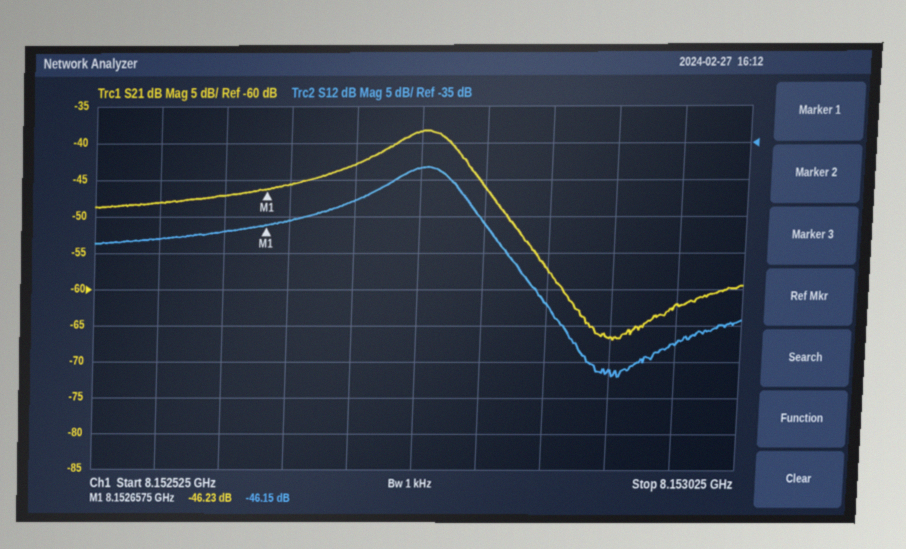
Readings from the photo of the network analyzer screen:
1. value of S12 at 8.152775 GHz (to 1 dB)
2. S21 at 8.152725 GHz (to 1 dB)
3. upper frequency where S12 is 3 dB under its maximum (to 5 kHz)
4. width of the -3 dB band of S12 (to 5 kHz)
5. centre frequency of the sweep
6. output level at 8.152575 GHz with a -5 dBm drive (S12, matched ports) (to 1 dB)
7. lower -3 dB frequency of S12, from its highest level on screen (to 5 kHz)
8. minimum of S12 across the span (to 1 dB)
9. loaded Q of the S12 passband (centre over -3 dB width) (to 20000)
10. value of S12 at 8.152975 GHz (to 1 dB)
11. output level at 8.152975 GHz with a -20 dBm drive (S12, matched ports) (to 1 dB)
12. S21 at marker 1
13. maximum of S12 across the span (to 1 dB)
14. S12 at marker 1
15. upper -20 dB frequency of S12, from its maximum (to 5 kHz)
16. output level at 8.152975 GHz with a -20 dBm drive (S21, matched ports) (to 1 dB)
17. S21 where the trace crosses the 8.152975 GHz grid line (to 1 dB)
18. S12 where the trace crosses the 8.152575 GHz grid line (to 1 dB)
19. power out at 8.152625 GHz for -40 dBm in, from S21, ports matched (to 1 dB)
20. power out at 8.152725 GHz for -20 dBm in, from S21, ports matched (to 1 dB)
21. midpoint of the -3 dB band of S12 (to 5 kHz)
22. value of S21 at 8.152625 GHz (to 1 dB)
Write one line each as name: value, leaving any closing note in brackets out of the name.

value of S12 at 8.152775 GHz: -38 dB
S21 at 8.152725 GHz: -43 dB
upper frequency where S12 is 3 dB under its maximum: 8.152805 GHz
width of the -3 dB band of S12: 60 kHz
centre frequency of the sweep: 8.152775 GHz
output level at 8.152575 GHz with a -5 dBm drive (S12, matched ports): -53 dBm
lower -3 dB frequency of S12, from its highest level on screen: 8.152745 GHz
minimum of S12 across the span: -67 dB
loaded Q of the S12 passband (centre over -3 dB width): 140000
value of S12 at 8.152975 GHz: -63 dB
output level at 8.152975 GHz with a -20 dBm drive (S12, matched ports): -83 dBm
S21 at marker 1: -46.23 dB
maximum of S12 across the span: -38 dB
S12 at marker 1: -46.15 dB
upper -20 dB frequency of S12, from its maximum: 8.152880 GHz
output level at 8.152975 GHz with a -20 dBm drive (S21, matched ports): -82 dBm
S21 where the trace crosses the 8.152975 GHz grid line: -62 dB
S12 where the trace crosses the 8.152575 GHz grid line: -48 dB
power out at 8.152625 GHz for -40 dBm in, from S21, ports matched: -87 dBm
power out at 8.152725 GHz for -20 dBm in, from S21, ports matched: -63 dBm
midpoint of the -3 dB band of S12: 8.152775 GHz
value of S21 at 8.152625 GHz: -47 dB
